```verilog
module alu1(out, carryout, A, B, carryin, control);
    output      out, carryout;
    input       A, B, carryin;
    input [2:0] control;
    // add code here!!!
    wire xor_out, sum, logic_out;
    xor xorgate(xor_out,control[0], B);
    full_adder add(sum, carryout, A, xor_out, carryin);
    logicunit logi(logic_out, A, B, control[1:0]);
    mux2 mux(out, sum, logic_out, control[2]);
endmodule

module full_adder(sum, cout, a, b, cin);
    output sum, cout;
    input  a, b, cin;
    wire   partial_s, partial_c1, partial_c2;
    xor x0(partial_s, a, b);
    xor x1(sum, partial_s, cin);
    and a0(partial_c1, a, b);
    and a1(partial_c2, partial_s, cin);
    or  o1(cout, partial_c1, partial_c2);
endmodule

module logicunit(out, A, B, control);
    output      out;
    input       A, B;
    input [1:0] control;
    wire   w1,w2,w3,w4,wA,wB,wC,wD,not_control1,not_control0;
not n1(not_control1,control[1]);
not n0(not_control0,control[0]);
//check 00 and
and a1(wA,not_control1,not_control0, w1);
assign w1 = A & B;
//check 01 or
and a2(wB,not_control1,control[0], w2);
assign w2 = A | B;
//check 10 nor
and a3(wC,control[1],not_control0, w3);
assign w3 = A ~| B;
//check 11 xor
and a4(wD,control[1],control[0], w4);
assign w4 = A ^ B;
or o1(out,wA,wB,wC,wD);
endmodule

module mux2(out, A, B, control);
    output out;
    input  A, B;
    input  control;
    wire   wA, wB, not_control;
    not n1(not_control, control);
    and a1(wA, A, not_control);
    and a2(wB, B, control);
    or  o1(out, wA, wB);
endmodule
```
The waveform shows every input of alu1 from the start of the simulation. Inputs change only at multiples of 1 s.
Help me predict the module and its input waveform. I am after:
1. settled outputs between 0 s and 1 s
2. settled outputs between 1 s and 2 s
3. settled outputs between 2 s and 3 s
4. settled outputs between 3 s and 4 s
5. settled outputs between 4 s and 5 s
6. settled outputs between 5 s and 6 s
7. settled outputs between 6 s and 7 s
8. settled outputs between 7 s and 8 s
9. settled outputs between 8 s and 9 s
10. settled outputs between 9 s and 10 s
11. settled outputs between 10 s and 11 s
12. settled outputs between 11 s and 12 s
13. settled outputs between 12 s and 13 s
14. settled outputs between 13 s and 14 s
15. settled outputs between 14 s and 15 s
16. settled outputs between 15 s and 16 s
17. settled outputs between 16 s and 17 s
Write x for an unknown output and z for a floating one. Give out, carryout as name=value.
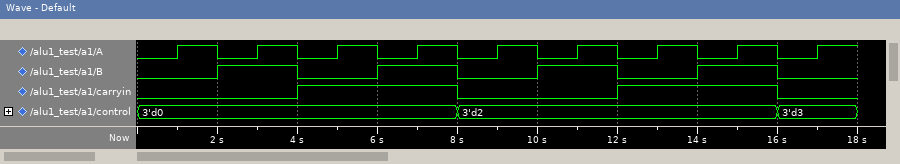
out=0, carryout=0
out=1, carryout=0
out=1, carryout=0
out=0, carryout=1
out=1, carryout=0
out=0, carryout=1
out=0, carryout=1
out=1, carryout=1
out=0, carryout=0
out=1, carryout=0
out=1, carryout=0
out=0, carryout=1
out=1, carryout=0
out=0, carryout=1
out=0, carryout=1
out=1, carryout=1
out=1, carryout=0
